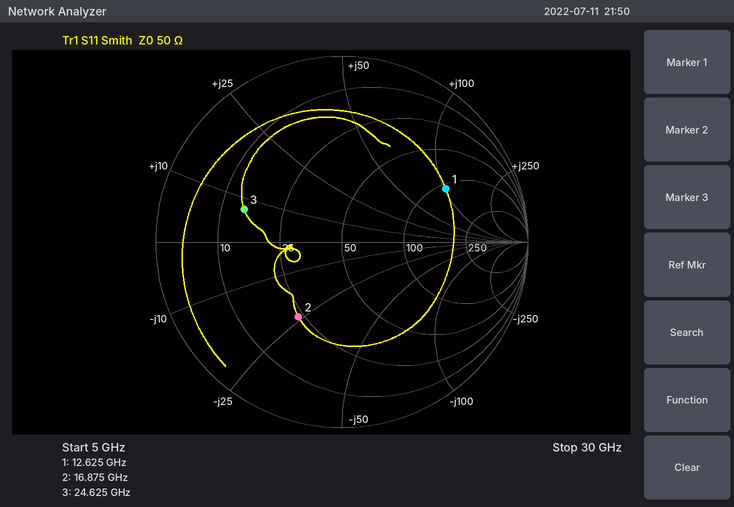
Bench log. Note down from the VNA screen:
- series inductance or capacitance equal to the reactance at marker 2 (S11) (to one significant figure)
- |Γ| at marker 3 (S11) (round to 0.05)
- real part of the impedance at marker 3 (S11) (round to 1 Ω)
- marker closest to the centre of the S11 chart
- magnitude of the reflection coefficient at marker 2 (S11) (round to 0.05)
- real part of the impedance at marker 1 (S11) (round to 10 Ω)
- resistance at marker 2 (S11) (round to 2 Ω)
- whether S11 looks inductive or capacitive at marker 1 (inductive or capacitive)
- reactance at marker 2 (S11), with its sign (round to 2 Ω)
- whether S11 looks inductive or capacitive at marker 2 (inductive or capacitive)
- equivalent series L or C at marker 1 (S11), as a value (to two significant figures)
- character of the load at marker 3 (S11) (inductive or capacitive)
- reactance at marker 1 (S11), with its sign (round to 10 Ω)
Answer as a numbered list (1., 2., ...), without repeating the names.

1. 400 fF
2. 0.55
3. 15 Ω
4. marker 2
5. 0.45
6. 110 Ω
7. 24 Ω
8. inductive
9. -24 Ω
10. capacitive
11. 1.3 nH
12. inductive
13. +100 Ω
